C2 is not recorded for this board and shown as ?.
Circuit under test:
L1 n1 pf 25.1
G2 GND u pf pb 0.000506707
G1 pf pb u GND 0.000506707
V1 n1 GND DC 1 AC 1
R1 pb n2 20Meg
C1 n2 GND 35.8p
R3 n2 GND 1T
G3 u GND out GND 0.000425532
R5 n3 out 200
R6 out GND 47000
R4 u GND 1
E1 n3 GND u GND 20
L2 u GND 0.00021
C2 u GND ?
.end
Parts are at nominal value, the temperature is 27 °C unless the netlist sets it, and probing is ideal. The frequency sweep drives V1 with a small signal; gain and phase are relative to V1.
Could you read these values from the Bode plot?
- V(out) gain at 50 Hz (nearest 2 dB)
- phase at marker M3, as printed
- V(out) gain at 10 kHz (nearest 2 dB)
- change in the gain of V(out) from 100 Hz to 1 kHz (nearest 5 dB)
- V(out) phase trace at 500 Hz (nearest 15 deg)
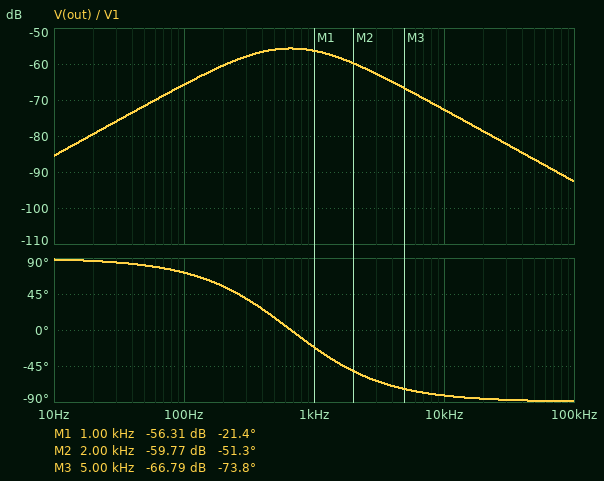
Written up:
-72 dB
-73.8 deg
-72 dB
10 dB
15 deg
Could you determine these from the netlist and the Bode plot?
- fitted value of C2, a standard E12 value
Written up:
680 µF
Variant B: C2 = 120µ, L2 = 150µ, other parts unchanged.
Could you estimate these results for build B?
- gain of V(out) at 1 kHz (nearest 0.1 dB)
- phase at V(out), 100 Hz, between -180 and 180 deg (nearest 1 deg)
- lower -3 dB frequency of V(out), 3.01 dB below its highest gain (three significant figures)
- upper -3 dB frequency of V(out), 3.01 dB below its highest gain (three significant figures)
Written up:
-55.9 dB
74 deg
343 Hz
8.08 kHz
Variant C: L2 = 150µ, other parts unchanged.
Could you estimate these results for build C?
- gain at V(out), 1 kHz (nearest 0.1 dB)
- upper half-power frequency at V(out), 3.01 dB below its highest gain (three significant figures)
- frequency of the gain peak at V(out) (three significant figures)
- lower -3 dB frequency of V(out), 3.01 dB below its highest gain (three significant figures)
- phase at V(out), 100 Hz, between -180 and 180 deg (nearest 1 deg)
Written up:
-56.2 dB
1.72 kHz
715 Hz
297 Hz
74 deg
